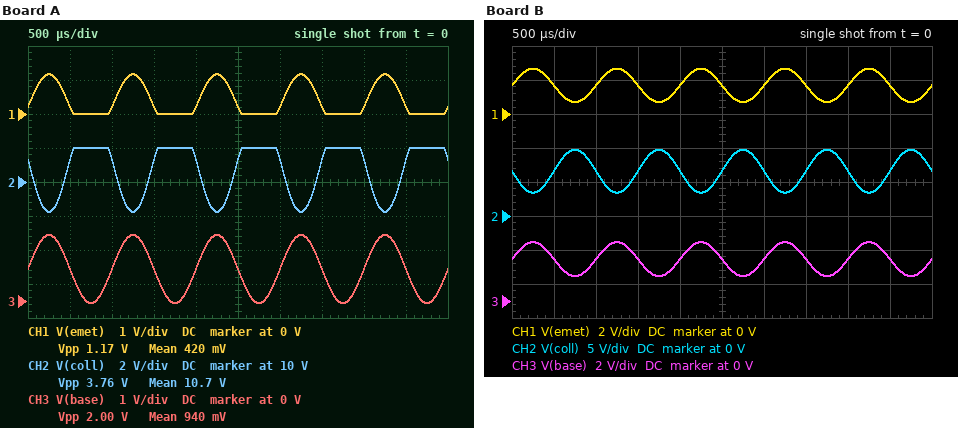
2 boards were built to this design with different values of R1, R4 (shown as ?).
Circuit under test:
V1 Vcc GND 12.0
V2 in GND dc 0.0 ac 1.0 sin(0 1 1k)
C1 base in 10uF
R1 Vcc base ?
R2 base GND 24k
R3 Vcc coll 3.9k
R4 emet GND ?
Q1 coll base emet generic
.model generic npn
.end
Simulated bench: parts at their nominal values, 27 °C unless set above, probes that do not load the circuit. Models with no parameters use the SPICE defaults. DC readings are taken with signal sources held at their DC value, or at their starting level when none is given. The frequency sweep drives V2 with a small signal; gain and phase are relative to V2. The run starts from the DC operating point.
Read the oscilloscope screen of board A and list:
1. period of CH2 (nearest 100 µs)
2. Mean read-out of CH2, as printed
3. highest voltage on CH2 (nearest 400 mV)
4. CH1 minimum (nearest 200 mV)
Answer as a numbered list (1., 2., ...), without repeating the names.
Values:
1. 1.0 ms
2. 10.7 V
3. 12.0 V
4. 0 V
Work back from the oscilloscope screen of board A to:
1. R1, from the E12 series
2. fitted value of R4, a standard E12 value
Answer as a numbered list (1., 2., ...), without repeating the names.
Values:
1. 270 kΩ
2. 1.2 kΩ
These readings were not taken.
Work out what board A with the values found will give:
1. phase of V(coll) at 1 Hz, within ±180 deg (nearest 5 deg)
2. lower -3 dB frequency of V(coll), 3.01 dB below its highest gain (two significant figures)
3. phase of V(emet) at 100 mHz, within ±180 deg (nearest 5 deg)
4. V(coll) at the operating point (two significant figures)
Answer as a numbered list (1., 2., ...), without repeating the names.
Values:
1. -140 deg
2. 840 mHz
3. 85 deg
4. 11 V
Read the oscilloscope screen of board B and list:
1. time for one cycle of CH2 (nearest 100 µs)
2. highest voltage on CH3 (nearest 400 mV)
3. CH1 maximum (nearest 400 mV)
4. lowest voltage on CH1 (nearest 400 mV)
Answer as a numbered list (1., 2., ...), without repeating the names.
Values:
1. 1.0 ms
2. 3.6 V
3. 2.8 V
4. 800 mV
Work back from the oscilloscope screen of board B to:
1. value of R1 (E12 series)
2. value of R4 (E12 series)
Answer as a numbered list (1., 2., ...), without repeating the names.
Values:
1. 82 kΩ
2. 1.2 kΩ
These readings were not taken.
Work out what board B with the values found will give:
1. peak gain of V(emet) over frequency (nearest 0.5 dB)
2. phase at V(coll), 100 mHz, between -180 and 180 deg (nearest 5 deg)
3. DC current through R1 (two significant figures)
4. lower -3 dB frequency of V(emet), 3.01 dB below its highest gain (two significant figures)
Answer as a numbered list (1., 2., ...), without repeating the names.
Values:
1. 0 dB
2. -95 deg
3. 120 µA
4. 990 mHz
